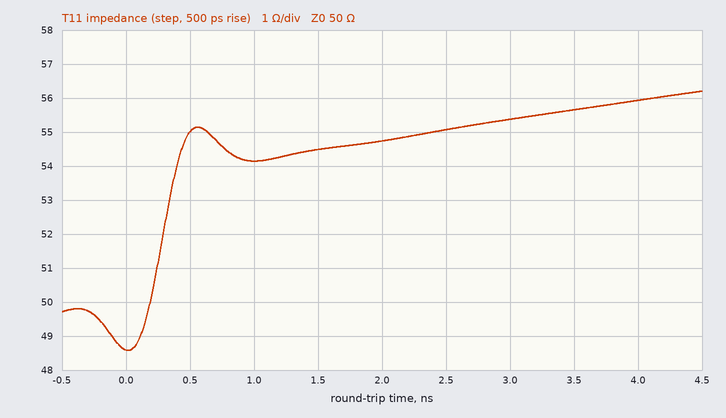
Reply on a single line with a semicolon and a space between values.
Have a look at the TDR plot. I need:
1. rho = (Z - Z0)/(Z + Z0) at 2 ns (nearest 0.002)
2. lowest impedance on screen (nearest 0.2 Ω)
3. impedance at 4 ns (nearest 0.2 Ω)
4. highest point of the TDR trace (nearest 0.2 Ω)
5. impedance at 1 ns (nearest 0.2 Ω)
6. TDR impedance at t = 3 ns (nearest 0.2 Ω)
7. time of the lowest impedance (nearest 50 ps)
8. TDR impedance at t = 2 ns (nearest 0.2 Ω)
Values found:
+0.046; 48.6 Ω; 56.0 Ω; 56.2 Ω; 54.2 Ω; 55.4 Ω; 0 ps; 54.8 Ω
